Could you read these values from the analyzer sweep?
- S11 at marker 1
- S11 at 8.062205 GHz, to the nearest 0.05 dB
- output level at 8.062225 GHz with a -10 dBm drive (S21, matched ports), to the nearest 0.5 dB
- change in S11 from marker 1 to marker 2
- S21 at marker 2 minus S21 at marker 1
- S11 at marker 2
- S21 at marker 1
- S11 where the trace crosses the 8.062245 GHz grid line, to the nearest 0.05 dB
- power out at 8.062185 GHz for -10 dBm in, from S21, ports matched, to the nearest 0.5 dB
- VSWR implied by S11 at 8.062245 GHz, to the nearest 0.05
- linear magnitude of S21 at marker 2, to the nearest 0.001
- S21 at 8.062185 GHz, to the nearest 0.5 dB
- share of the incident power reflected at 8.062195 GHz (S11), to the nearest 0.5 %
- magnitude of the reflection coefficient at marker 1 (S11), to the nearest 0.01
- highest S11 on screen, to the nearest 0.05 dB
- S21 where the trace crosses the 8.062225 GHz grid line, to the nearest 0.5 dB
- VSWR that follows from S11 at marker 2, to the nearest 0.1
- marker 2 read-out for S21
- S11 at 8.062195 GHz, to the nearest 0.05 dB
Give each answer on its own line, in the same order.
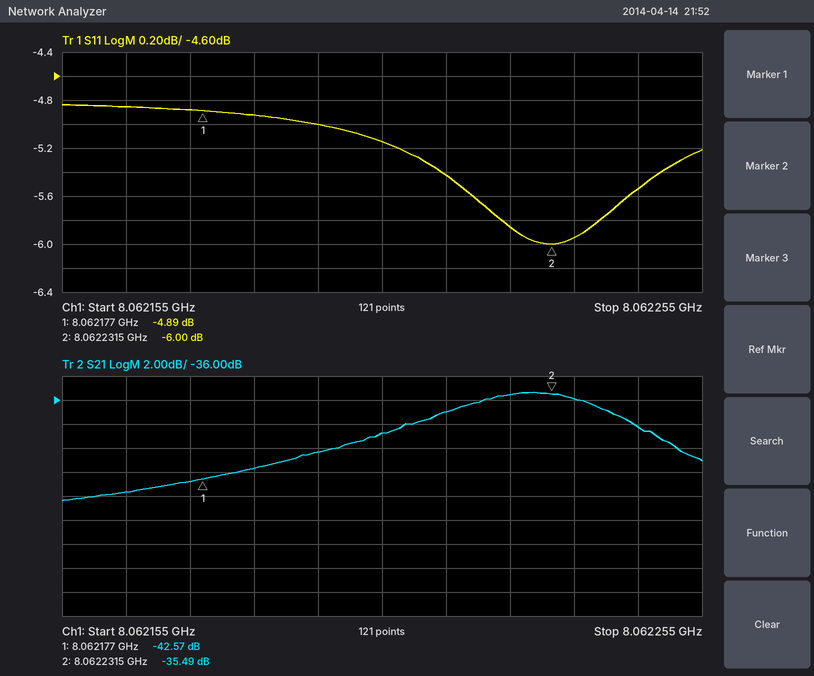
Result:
-4.89 dB
-5.15 dB
-45.5 dBm
-1.11 dB
7.08 dB
-6.00 dB
-42.57 dB
-5.55 dB
-51.5 dBm
3.25
0.017
-41.5 dB
31.5 %
0.57
-4.85 dB
-35.5 dB
3.0
-35.49 dB
-5.00 dB
